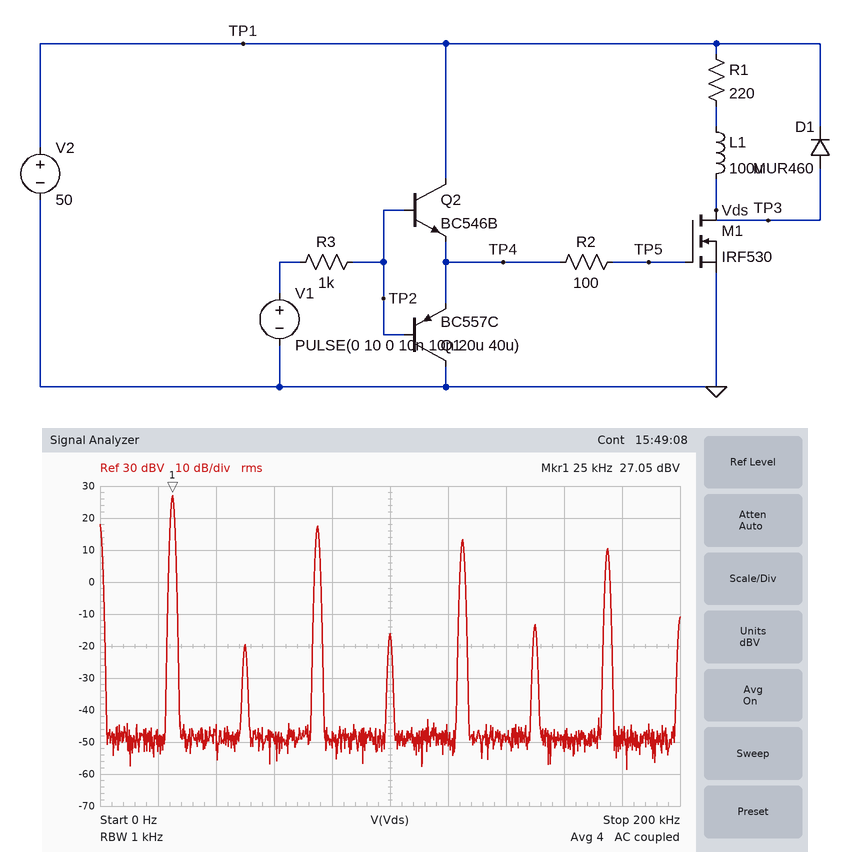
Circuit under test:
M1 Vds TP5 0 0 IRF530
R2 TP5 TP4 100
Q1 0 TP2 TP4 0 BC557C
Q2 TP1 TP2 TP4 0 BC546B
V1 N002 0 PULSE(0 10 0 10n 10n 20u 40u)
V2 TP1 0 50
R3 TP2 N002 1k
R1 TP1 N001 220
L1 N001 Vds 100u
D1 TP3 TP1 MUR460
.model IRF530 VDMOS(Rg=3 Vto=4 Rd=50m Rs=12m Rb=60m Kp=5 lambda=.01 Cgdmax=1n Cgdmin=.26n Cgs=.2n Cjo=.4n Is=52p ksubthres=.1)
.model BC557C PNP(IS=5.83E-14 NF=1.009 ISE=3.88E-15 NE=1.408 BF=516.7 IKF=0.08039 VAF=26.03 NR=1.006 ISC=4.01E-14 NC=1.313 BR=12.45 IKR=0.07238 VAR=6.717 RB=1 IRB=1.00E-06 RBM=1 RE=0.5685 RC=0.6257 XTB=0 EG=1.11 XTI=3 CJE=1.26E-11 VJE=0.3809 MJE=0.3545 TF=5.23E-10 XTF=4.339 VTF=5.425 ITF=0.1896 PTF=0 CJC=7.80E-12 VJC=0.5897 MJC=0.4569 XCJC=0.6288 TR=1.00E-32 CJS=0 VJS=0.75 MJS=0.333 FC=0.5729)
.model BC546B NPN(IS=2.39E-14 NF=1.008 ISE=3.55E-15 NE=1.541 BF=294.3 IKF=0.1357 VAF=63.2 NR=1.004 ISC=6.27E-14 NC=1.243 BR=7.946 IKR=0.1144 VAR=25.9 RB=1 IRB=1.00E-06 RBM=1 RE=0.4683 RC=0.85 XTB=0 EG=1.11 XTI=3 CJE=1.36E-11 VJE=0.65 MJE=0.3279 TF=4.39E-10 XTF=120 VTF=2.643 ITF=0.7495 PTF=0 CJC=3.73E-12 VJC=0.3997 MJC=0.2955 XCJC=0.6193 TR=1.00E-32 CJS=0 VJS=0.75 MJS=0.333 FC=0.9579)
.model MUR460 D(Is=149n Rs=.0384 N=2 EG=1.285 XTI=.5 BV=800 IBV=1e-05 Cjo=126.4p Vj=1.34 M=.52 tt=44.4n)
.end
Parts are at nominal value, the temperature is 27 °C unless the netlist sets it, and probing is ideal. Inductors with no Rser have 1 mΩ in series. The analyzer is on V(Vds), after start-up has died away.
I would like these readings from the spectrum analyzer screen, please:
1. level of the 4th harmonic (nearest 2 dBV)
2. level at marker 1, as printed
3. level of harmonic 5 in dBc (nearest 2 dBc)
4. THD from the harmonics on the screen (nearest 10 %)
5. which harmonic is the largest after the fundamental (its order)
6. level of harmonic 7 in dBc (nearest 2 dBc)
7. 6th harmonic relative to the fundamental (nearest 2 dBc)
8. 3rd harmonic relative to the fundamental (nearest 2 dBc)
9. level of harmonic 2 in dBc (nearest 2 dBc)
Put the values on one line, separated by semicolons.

-16 dBV; 27.05 dBV; -14 dBc; 40 %; 3; -16 dBc; -40 dBc; -10 dBc; -46 dBc
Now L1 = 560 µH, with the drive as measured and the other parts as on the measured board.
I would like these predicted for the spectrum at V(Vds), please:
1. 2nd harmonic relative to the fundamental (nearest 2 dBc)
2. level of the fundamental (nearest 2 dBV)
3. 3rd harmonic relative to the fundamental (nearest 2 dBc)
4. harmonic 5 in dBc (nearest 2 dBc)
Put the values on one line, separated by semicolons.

-18 dBc; 28 dBV; -8 dBc; -10 dBc
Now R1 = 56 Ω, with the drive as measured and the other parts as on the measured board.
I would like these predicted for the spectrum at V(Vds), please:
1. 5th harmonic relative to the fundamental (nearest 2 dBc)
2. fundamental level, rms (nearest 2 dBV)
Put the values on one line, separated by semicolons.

-12 dBc; 28 dBV
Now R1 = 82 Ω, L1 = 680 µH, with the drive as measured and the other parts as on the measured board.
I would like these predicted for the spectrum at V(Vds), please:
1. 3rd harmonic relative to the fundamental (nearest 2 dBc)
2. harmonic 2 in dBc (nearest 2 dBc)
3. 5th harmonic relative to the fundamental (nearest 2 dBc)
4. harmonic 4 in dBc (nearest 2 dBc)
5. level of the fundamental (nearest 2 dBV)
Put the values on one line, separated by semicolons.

-4 dBc; -8 dBc; -4 dBc; -6 dBc; 28 dBV
